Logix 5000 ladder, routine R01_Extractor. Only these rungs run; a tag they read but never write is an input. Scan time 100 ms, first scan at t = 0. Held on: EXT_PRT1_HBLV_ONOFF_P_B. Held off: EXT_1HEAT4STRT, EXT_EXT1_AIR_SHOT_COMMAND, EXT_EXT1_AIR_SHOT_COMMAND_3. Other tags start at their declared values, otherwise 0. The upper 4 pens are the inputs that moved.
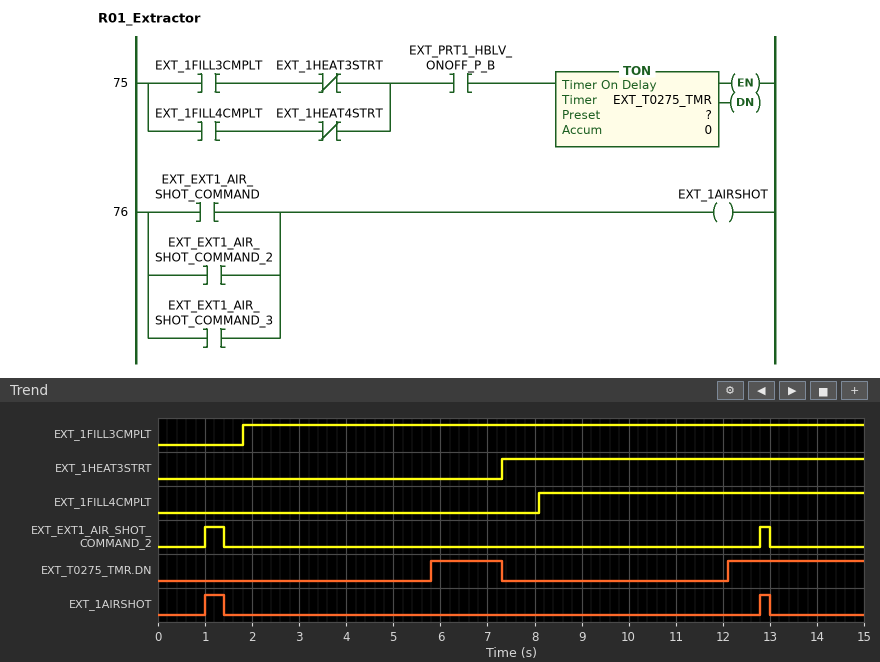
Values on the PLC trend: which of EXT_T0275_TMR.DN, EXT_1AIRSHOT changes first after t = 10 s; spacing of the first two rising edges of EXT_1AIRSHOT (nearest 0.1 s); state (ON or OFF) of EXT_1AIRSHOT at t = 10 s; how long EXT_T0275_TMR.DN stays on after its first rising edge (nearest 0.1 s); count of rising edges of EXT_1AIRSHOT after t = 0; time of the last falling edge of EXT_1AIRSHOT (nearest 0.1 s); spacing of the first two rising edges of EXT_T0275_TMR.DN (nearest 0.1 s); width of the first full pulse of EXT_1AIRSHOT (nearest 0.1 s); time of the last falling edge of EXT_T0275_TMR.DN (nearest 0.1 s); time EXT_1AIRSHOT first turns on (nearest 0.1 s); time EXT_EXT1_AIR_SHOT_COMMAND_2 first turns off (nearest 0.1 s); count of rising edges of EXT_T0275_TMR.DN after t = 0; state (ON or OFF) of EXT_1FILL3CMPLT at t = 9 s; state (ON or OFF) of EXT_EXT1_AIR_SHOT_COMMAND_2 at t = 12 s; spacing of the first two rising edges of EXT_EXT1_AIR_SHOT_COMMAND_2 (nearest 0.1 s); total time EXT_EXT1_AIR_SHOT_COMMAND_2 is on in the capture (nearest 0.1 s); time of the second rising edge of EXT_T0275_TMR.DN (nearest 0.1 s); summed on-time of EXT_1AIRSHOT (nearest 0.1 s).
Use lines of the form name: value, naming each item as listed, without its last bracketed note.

which of EXT_T0275_TMR.DN, EXT_1AIRSHOT changes first after t = 10 s: EXT_T0275_TMR.DN
spacing of the first two rising edges of EXT_1AIRSHOT: 11.8 s
state (ON or OFF) of EXT_1AIRSHOT at t = 10 s: OFF
how long EXT_T0275_TMR.DN stays on after its first rising edge: 1.5 s
count of rising edges of EXT_1AIRSHOT after t = 0: 2
time of the last falling edge of EXT_1AIRSHOT: 13.0 s
spacing of the first two rising edges of EXT_T0275_TMR.DN: 6.3 s
width of the first full pulse of EXT_1AIRSHOT: 0.4 s
time of the last falling edge of EXT_T0275_TMR.DN: 7.3 s
time EXT_1AIRSHOT first turns on: 1.0 s
time EXT_EXT1_AIR_SHOT_COMMAND_2 first turns off: 1.4 s
count of rising edges of EXT_T0275_TMR.DN after t = 0: 2
state (ON or OFF) of EXT_1FILL3CMPLT at t = 9 s: ON
state (ON or OFF) of EXT_EXT1_AIR_SHOT_COMMAND_2 at t = 12 s: OFF
spacing of the first two rising edges of EXT_EXT1_AIR_SHOT_COMMAND_2: 11.8 s
total time EXT_EXT1_AIR_SHOT_COMMAND_2 is on in the capture: 0.6 s
time of the second rising edge of EXT_T0275_TMR.DN: 12.1 s
summed on-time of EXT_1AIRSHOT: 0.6 s
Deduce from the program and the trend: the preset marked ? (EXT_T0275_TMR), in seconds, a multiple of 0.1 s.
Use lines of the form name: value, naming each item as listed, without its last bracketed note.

the preset marked ? (EXT_T0275_TMR), in seconds, a multiple of 0.1 s: 4.0 s
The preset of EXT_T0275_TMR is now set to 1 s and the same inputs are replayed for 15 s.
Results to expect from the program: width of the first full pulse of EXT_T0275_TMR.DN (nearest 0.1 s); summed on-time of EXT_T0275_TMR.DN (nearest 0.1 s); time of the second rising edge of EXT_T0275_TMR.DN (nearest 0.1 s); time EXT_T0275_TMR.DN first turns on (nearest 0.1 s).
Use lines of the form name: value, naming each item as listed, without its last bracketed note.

width of the first full pulse of EXT_T0275_TMR.DN: 4.5 s
summed on-time of EXT_T0275_TMR.DN: 10.4 s
time of the second rising edge of EXT_T0275_TMR.DN: 9.1 s
time EXT_T0275_TMR.DN first turns on: 2.8 s
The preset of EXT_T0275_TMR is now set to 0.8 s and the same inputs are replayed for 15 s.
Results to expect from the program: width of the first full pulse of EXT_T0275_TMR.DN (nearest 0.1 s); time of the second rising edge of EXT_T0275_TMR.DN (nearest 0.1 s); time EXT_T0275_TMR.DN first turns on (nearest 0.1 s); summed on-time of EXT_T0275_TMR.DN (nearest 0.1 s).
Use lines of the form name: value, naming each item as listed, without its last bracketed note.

width of the first full pulse of EXT_T0275_TMR.DN: 4.7 s
time of the second rising edge of EXT_T0275_TMR.DN: 8.9 s
time EXT_T0275_TMR.DN first turns on: 2.6 s
summed on-time of EXT_T0275_TMR.DN: 10.8 s
